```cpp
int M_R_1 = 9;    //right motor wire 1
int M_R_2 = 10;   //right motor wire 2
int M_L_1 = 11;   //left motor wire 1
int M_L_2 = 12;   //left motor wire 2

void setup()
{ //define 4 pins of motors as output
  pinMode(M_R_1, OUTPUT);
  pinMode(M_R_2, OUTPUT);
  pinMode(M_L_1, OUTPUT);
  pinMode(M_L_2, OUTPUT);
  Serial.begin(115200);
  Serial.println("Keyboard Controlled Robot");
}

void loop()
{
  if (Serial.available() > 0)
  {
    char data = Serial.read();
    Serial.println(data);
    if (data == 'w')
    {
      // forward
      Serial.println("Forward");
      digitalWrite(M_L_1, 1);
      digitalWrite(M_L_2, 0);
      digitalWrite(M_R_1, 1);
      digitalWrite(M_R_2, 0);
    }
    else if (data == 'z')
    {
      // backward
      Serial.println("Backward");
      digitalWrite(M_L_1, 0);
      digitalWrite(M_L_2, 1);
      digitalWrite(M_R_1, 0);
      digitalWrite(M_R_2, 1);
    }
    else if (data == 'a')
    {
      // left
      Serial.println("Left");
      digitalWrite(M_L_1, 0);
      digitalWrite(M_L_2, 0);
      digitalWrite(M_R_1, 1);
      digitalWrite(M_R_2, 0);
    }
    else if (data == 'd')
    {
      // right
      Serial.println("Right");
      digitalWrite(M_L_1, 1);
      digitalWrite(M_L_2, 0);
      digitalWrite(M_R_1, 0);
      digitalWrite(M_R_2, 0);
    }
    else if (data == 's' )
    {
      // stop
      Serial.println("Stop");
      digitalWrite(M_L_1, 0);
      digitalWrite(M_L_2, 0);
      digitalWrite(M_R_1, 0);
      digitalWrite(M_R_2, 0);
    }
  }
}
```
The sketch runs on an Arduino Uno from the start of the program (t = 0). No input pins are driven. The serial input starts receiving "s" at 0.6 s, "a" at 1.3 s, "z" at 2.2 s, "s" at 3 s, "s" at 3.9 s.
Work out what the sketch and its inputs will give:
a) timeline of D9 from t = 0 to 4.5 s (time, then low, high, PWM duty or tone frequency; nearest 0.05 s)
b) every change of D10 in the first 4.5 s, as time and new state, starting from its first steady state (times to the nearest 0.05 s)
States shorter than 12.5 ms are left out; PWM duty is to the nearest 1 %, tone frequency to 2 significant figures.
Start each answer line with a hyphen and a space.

- 0 s low; 1.3 s high; 2.2 s low
- 0 s low; 2.2 s high; 3 s low
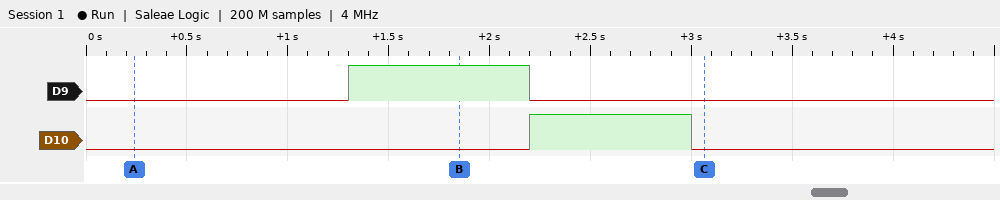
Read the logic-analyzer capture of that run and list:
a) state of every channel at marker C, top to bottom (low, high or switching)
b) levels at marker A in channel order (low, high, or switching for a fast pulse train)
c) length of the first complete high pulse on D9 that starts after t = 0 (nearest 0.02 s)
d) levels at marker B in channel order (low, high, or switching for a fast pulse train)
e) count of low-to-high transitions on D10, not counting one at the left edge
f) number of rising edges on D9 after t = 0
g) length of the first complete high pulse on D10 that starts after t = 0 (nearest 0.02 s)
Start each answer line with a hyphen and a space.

- D9 low, D10 low
- D9 low, D10 low
- 0.90 s
- D9 high, D10 low
- 1
- 1
- 0.80 s
